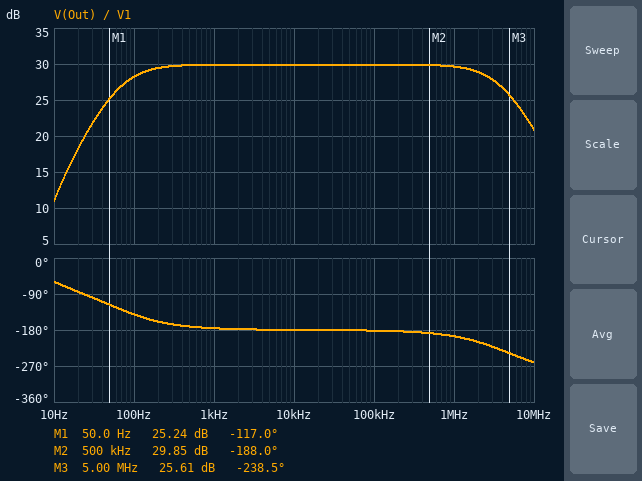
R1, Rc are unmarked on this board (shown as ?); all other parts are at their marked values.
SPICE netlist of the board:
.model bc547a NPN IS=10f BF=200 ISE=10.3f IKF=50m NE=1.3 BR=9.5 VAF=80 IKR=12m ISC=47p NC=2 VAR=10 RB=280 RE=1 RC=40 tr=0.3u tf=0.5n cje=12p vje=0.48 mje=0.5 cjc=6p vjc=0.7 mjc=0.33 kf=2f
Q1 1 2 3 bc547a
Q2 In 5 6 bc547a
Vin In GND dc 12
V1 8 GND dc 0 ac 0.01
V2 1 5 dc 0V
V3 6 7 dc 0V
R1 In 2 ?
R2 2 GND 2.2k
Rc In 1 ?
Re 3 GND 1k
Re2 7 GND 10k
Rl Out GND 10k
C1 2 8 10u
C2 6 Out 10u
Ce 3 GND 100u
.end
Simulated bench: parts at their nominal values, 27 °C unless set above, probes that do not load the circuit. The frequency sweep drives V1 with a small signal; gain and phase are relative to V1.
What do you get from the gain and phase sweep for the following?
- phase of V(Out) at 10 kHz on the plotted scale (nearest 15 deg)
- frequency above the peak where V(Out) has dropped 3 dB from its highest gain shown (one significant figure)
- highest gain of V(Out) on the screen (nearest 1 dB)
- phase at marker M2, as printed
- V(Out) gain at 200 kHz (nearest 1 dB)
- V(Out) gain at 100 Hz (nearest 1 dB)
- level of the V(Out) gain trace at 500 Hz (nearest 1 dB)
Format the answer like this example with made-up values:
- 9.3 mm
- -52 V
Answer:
- -180 deg
- 4 MHz
- 30 dB
- -188.0 deg
- 30 dB
- 28 dB
- 30 dB
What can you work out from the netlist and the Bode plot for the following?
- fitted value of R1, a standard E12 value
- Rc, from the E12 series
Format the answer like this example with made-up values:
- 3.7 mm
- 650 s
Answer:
- 12 kΩ
- 820 Ω
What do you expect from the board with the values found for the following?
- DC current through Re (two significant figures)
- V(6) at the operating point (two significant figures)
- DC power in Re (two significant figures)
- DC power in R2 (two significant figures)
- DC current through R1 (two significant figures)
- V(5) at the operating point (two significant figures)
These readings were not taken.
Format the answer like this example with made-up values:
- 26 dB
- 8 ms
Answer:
- 1.2 mA
- 10 V
- 1.4 mW
- 1.5 mW
- 850 µA
- 11 V
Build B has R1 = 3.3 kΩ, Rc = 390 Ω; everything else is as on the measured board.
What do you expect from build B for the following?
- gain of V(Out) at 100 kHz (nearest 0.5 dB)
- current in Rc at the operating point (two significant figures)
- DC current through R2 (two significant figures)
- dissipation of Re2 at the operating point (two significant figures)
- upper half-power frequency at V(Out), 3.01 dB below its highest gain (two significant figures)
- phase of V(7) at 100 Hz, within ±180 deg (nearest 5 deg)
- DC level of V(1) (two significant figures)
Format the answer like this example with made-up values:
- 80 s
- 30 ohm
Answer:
- 31.5 dB
- 4.0 mA
- 2.2 mA
- 9.5 mW
- 2.8 MHz
- -115 deg
- 10 V
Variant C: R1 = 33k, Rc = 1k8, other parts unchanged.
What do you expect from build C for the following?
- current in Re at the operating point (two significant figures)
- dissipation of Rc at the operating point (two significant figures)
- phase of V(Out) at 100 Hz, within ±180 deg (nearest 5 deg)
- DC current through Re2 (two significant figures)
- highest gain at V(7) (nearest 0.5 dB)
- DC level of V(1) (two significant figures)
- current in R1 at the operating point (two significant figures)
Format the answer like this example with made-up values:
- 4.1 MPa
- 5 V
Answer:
- 140 µA
- 42 µW
- -170 deg
- 1.1 mA
- 19.5 dB
- 12 V
- 340 µA
